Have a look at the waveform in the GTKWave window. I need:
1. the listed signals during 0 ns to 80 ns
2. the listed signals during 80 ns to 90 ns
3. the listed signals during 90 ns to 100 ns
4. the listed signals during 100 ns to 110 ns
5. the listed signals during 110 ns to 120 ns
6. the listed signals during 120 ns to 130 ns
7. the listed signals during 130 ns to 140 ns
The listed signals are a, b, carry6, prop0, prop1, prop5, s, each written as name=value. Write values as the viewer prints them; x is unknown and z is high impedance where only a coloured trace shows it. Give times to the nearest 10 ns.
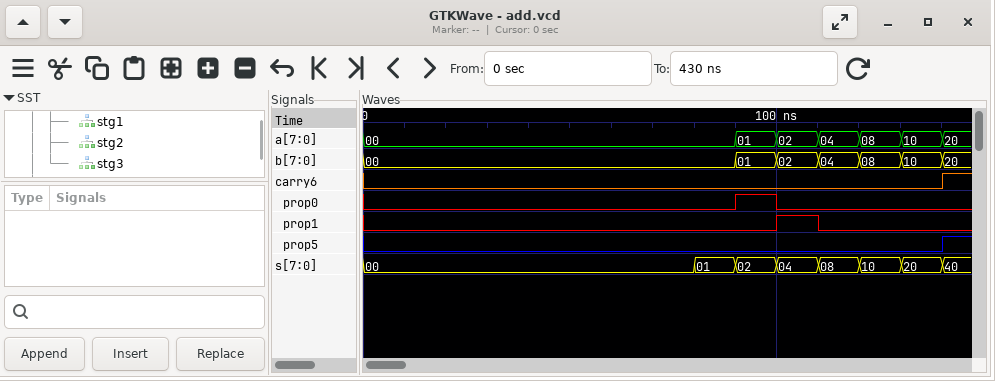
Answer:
a=00, b=00, carry6=0, prop0=0, prop1=0, prop5=0, s=00
a=00, b=00, carry6=0, prop0=0, prop1=0, prop5=0, s=01
a=01, b=01, carry6=0, prop0=1, prop1=0, prop5=0, s=02
a=02, b=02, carry6=0, prop0=0, prop1=1, prop5=0, s=04
a=04, b=04, carry6=0, prop0=0, prop1=0, prop5=0, s=08
a=08, b=08, carry6=0, prop0=0, prop1=0, prop5=0, s=10
a=10, b=10, carry6=0, prop0=0, prop1=0, prop5=0, s=20
